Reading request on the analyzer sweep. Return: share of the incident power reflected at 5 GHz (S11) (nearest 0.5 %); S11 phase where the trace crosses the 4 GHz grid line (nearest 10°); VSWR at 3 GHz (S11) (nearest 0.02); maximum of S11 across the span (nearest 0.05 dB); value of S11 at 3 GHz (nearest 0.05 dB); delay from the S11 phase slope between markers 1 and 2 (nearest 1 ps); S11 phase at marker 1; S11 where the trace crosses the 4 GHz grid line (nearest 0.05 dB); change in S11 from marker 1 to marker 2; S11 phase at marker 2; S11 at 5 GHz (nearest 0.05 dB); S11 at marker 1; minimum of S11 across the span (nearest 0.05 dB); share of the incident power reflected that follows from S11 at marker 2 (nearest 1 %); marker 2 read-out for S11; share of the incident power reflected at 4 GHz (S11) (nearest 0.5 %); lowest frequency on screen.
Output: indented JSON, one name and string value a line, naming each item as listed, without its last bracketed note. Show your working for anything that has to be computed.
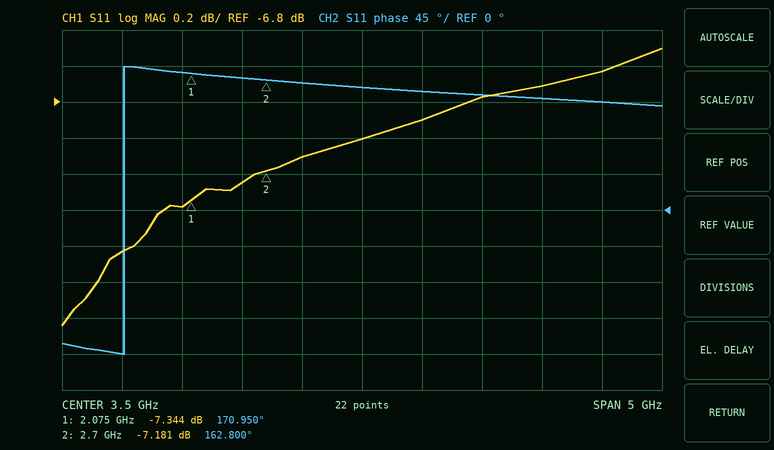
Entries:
{
  "share of the incident power reflected at 5 GHz (S11)": "10^(-6.7/10) ≈ 21.4 %, so 21.5 % to the nearest 0.5 %",
  "S11 phase where the trace crosses the 4 GHz grid line": "150°",
  "VSWR at 3 GHz (S11)": "|Γ| = 10^(-7.1/20) = 0.4416; VSWR = (1 + 0.4416)/(1 − 0.4416) ≈ 2.58",
  "maximum of S11 across the span": "-6.50 dB",
  "value of S11 at 3 GHz": "-7.10 dB",
  "delay from the S11 phase slope between markers 1 and 2": "−(162.8° − (170.95°))/(360° × 625 MHz) ≈ 36 ps",
  "S11 phase at marker 1": "170.950°",
  "S11 where the trace crosses the 4 GHz grid line": "-6.90 dB",
  "change in S11 from marker 1 to marker 2": "-7.181 − (-7.344) = 0.163 dB",
  "S11 phase at marker 2": "162.800°",
  "S11 at 5 GHz": "-6.70 dB",
  "S11 at marker 1": "-7.344 dB",
  "minimum of S11 across the span": "-8.05 dB",
  "share of the incident power reflected that follows from S11 at marker 2": "10^(-7.181/10) ≈ 19 %",
  "marker 2 read-out for S11": "-7.181 dB",
  "share of the incident power reflected at 4 GHz (S11)": "10^(-6.9/10) ≈ 20.4 %, so 20.5 % to the nearest 0.5 %",
  "lowest frequency on screen": "1 GHz"
}
